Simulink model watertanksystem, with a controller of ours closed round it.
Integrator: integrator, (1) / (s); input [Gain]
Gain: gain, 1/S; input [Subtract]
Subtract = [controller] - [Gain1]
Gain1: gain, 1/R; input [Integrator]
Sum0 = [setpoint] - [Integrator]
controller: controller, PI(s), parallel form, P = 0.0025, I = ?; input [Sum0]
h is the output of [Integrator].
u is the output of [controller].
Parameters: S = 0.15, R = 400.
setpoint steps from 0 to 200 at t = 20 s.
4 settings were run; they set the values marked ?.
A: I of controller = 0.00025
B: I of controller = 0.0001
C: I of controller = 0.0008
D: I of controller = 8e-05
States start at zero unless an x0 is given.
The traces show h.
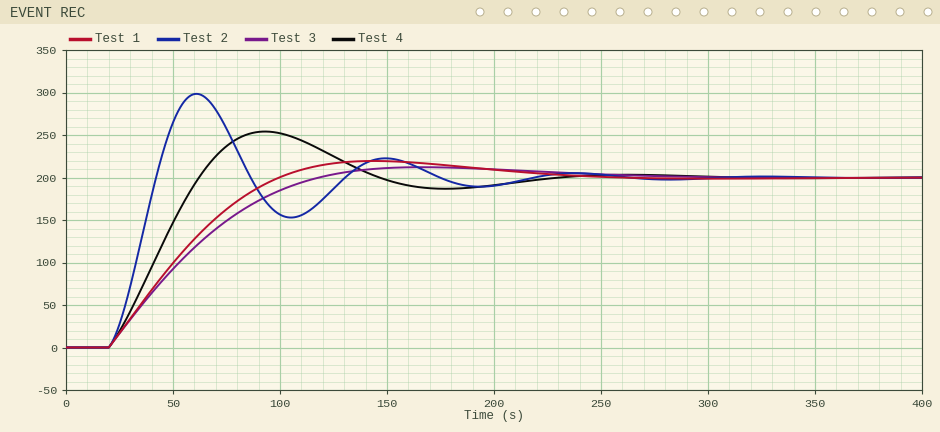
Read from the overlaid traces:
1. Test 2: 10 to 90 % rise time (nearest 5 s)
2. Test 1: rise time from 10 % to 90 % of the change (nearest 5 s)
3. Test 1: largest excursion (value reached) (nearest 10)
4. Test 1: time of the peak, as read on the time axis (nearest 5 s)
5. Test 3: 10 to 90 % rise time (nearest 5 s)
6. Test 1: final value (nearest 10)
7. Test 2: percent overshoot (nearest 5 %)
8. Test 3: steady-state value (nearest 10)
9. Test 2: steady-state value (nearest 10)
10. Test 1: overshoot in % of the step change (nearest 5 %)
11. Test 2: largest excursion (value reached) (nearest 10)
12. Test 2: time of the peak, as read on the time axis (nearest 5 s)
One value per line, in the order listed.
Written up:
15 s
60 s
220
145 s
70 s
200
50 %
200
200
10 %
300
60 s
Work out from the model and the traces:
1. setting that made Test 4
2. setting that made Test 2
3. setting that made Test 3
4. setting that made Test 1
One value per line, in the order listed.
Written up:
A
C
D
B
